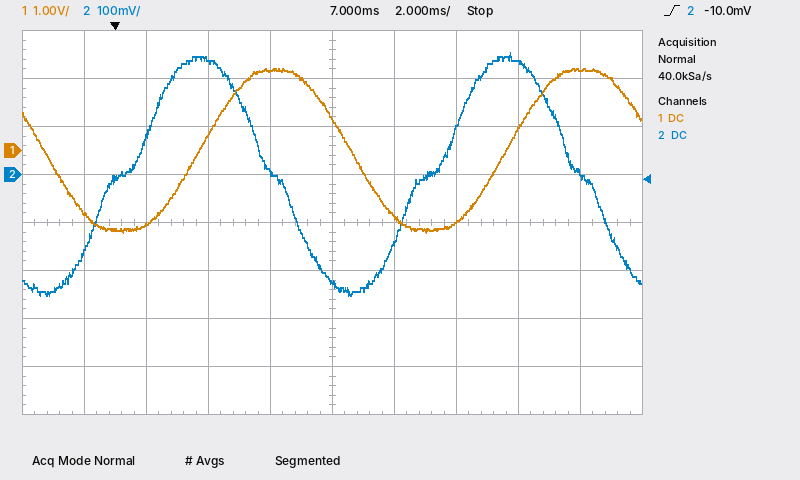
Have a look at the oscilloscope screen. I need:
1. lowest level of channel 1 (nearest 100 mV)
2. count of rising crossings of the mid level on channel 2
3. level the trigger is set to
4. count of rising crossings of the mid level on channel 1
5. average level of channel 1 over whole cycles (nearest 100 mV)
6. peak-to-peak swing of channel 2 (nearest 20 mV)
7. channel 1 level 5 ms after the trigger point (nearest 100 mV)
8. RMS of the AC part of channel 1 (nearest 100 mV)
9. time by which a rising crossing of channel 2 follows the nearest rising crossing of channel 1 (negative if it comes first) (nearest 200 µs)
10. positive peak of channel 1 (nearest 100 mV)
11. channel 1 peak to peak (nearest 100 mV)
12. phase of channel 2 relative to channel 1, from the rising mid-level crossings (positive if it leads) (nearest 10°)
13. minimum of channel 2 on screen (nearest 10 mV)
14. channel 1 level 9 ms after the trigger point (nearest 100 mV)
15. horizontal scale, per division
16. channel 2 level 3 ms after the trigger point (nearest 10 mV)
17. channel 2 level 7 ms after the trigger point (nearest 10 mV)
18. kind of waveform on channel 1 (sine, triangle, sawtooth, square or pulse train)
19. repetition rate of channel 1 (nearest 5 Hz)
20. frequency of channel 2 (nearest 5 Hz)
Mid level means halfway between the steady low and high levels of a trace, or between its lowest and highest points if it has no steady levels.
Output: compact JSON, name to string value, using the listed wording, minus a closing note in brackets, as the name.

{"lowest level of channel 1": "-1.7 V", "count of rising crossings of the mid level on channel 2": "2", "level the trigger is set to": "-10.0 mV", "count of rising crossings of the mid level on channel 1": "2", "average level of channel 1 over whole cycles": "0.0 V", "peak-to-peak swing of channel 2": "500 mV", "channel 1 level 5 ms after the trigger point": "1.7 V", "RMS of the AC part of channel 1": "1.2 V", "time by which a rising crossing of channel 2 follows the nearest rising crossing of channel 1 (negative if it comes first)": "-2.4 ms", "positive peak of channel 1": "1.7 V", "channel 1 peak to peak": "3.4 V", "phase of channel 2 relative to channel 1, from the rising mid-level crossings (positive if it leads)": "+90°", "minimum of channel 2 on screen": "-250 mV", "channel 1 level 9 ms after the trigger point": "-1.4 V", "horizontal scale, per division": "2 ms", "channel 2 level 3 ms after the trigger point": "240 mV", "channel 2 level 7 ms after the trigger point": "-230 mV", "kind of waveform on channel 1": "sine", "repetition rate of channel 1": "100 Hz", "frequency of channel 2": "100 Hz"}
